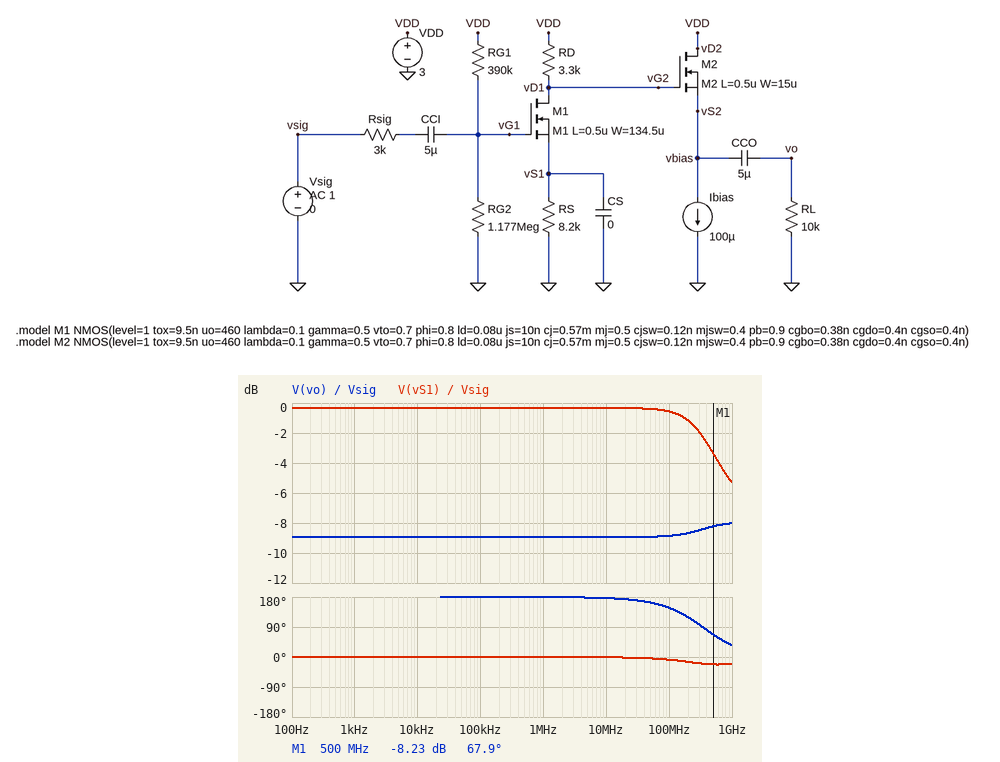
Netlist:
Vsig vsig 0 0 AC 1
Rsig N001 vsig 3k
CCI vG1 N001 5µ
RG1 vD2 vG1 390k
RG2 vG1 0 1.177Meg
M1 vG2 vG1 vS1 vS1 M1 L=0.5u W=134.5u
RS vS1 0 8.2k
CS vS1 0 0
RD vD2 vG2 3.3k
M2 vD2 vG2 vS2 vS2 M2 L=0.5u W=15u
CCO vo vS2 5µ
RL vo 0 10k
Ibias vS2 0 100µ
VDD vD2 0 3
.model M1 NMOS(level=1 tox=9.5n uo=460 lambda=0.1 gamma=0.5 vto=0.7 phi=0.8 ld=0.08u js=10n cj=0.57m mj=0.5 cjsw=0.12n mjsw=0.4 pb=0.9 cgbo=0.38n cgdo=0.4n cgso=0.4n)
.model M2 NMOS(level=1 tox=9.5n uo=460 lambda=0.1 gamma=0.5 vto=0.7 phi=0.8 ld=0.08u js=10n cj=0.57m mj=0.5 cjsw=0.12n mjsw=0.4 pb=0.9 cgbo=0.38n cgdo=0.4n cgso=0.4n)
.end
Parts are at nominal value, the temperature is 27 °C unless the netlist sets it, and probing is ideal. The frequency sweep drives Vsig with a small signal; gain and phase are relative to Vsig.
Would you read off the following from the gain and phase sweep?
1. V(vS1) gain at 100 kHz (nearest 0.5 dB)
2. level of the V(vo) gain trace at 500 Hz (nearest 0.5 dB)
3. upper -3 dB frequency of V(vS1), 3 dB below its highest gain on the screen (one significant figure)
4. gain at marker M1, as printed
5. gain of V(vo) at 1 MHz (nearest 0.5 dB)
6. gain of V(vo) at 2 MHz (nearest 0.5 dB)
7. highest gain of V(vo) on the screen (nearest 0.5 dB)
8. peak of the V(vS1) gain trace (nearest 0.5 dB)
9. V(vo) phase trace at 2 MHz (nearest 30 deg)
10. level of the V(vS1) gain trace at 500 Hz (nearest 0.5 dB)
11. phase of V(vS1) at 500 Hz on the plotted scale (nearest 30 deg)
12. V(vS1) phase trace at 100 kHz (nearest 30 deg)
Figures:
-0.5 dB
-9.0 dB
500 MHz
-8.23 dB
-9.0 dB
-9.0 dB
-8.0 dB
-0.5 dB
180 deg
-0.5 dB
0 deg
0 deg
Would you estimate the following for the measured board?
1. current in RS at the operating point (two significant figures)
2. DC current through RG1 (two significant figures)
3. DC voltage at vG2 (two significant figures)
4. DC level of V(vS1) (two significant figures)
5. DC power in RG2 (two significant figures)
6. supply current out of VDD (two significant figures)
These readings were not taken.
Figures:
180 µA
1.9 µA
2.4 V
1.5 V
4.3 µW
280 µA
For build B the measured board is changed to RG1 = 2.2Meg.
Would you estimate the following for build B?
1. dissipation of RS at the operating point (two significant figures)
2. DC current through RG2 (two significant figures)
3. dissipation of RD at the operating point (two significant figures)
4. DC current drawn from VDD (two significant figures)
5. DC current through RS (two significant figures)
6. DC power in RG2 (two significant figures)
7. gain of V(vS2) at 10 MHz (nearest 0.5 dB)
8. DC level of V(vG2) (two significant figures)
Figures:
12 µW
890 nA
4.9 µW
140 µA
38 µA
930 nW
-9.0 dB
2.9 V
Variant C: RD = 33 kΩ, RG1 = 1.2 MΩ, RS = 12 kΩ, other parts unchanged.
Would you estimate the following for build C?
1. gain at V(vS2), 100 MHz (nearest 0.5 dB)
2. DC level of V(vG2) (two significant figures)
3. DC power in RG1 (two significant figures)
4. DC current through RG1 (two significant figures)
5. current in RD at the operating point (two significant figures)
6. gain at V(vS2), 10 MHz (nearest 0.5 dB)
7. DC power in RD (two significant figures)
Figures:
3.0 dB
960 mV
1.9 µW
1.3 µA
62 µA
7.5 dB
130 µW
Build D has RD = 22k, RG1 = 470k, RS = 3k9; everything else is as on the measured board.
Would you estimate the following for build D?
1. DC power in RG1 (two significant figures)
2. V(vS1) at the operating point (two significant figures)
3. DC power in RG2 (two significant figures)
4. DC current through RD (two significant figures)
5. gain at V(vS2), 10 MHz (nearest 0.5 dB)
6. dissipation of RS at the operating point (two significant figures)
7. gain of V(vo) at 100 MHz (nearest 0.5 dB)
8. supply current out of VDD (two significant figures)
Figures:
1.6 µW
450 mV
3.9 µW
120 µA
-25.5 dB
52 µW
-9.0 dB
220 µA
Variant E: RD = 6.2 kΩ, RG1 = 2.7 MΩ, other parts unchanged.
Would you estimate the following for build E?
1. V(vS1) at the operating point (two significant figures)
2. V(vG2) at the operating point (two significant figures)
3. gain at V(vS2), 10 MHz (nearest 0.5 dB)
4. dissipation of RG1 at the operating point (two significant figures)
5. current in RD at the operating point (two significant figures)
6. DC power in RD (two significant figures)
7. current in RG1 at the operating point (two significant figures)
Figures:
190 mV
2.9 V
-3.5 dB
1.6 µW
23 µA
3.2 µW
770 nA
